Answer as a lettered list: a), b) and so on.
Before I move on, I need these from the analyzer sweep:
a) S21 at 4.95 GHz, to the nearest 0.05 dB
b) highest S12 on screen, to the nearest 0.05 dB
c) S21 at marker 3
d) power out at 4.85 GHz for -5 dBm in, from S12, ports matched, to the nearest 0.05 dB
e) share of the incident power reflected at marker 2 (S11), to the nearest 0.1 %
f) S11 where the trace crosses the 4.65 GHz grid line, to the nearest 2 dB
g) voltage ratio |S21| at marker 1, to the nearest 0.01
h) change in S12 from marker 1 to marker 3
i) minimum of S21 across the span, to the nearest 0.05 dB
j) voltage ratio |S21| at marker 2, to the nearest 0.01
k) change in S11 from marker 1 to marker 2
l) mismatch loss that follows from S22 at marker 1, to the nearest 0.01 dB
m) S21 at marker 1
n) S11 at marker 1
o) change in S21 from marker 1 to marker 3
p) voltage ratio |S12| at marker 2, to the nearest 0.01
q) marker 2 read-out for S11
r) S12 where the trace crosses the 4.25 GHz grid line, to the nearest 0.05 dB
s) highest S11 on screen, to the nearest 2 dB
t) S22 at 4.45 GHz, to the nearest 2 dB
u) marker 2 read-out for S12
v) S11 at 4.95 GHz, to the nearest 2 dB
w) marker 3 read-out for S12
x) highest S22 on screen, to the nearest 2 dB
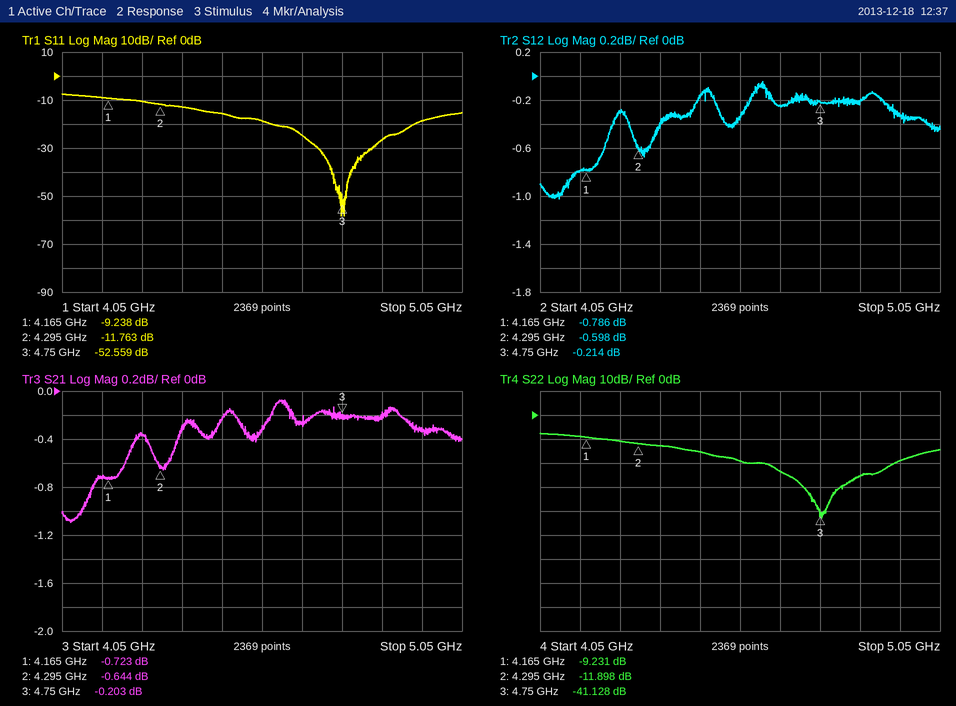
a) -0.30 dB
b) -0.05 dB
c) -0.203 dB
d) -5.20 dBm
e) 6.7 %
f) -24 dB
g) 0.92
h) 0.572 dB
i) -1.10 dB
j) 0.93
k) -2.525 dB
l) 0.55 dB
m) -0.723 dB
n) -9.238 dB
o) 0.520 dB
p) 0.93
q) -11.763 dB
r) -0.30 dB
s) -8 dB
t) -16 dB
u) -0.598 dB
v) -18 dB
w) -0.214 dB
x) -8 dB
